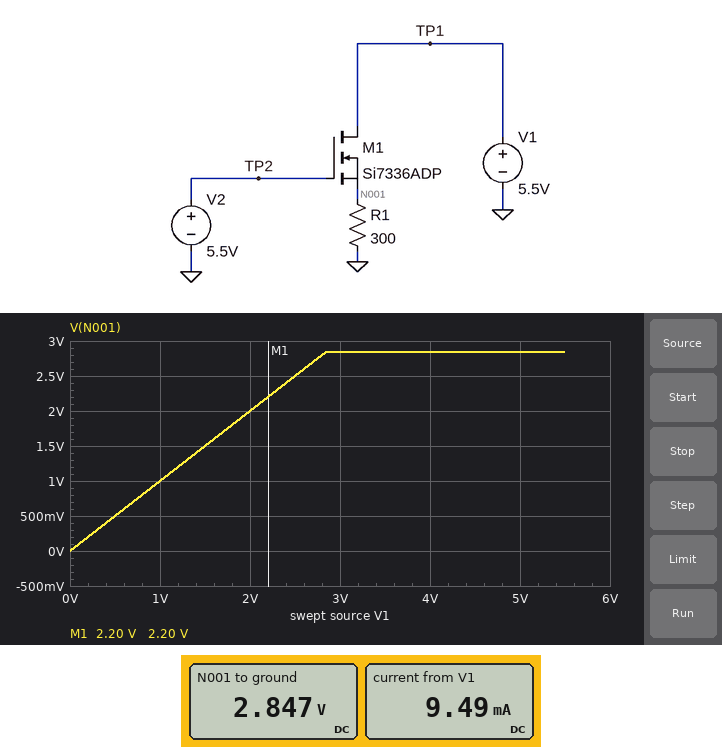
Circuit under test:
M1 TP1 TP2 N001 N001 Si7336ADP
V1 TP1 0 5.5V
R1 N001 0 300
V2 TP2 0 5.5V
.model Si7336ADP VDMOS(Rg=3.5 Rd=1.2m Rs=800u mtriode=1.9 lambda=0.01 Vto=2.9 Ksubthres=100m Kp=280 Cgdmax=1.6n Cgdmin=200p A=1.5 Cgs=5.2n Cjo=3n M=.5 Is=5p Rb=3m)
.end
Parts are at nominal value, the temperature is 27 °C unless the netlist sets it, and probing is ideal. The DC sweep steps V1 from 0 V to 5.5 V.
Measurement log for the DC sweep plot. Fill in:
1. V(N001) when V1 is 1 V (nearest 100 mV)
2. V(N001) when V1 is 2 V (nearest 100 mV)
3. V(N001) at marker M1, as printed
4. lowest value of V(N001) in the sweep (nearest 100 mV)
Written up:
1.0 V
2.0 V
2.20 V
0 V
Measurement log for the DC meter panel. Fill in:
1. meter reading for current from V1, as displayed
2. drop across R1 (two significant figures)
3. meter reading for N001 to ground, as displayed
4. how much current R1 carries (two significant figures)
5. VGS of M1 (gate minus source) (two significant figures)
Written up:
9.49 mA
2.8 V
2.847 V
9.5 mA
2.7 V
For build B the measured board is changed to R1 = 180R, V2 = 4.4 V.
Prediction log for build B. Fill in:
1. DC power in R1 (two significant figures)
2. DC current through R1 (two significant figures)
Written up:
17 mW
9.7 mA
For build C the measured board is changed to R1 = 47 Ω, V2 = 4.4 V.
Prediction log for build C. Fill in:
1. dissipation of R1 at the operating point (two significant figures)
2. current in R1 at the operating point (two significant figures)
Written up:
60 mW
36 mA
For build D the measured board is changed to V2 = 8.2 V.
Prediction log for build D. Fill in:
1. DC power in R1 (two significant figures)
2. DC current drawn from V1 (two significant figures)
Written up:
100 mW
18 mA
